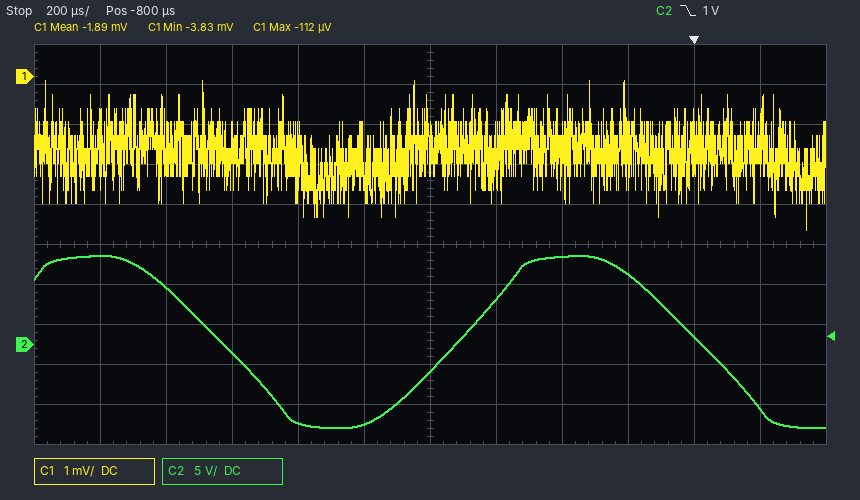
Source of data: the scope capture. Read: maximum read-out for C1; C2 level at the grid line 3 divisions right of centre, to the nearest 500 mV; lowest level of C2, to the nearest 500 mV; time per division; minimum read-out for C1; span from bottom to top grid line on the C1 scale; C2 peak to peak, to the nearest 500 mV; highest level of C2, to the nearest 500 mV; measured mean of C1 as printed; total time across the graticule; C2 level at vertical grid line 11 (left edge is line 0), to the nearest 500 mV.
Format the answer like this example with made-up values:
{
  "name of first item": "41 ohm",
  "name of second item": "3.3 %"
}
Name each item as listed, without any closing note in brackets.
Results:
{
  "maximum read-out for C1": "-112 µV",
  "C2 level at the grid line 3 divisions right of centre, to the nearest 500 mV": "9.0 V",
  "lowest level of C2, to the nearest 500 mV": "-10.5 V",
  "time per division": "200 µs",
  "minimum read-out for C1": "-3.83 mV",
  "span from bottom to top grid line on the C1 scale": "10 mV",
  "C2 peak to peak, to the nearest 500 mV": "21.5 V",
  "highest level of C2, to the nearest 500 mV": "11.0 V",
  "measured mean of C1 as printed": "-1.89 mV",
  "total time across the graticule": "2.4 ms",
  "C2 level at vertical grid line 11 (left edge is line 0), to the nearest 500 mV": "-8.0 V"
}
